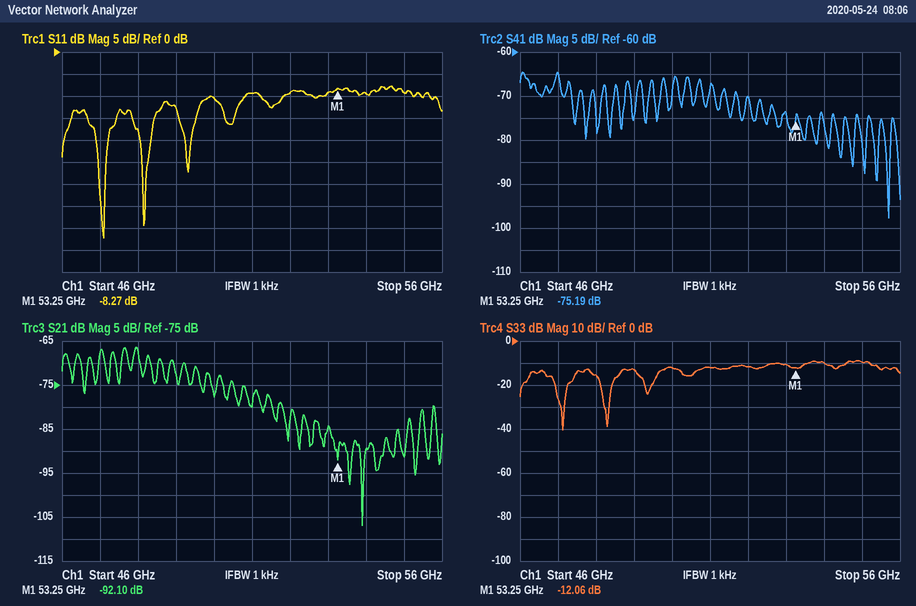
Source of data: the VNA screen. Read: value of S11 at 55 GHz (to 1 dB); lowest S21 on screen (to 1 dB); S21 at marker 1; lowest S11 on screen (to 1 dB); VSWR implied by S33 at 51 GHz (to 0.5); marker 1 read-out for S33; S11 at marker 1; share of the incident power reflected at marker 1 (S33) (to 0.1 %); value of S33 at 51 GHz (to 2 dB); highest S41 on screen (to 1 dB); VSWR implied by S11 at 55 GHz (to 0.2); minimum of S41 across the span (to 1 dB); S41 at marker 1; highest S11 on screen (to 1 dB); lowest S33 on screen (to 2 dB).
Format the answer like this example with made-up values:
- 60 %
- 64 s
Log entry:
- -9 dB
- -107 dB
- -92.10 dB
- -42 dB
- 1.5
- -12.06 dB
- -8.27 dB
- 6.2 %
- -12 dB
- -65 dB
- 2.0
- -98 dB
- -75.19 dB
- -8 dB
- -40 dB
